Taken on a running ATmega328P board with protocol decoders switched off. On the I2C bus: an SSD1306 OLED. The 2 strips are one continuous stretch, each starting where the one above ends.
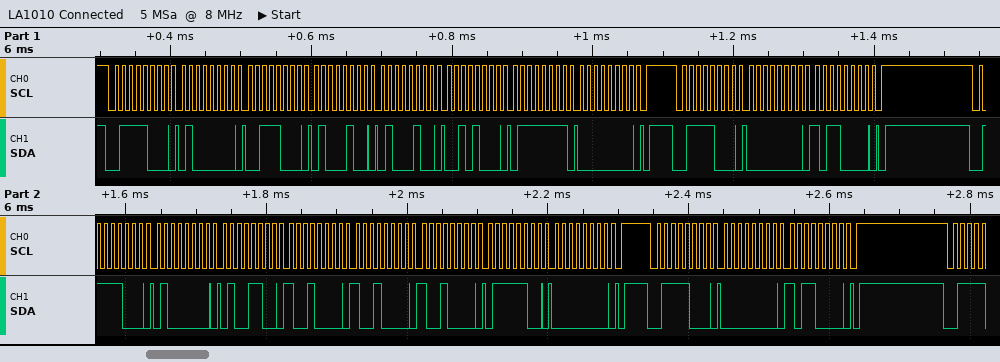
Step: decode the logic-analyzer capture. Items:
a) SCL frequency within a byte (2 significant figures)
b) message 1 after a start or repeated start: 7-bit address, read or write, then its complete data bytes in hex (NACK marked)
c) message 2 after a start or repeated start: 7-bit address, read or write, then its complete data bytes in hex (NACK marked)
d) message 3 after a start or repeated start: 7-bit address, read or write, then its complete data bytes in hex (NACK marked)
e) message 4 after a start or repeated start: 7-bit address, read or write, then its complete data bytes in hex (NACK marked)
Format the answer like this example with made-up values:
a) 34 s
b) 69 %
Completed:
a) 100 kHz
b) 0x3C write: 40 38 44 44 28 7F 00
c) 0x3C write: 00 B0
d) 0x3C write: 40 4C 90 90 90 7C 00
e) 0x3C write: 00 B0
